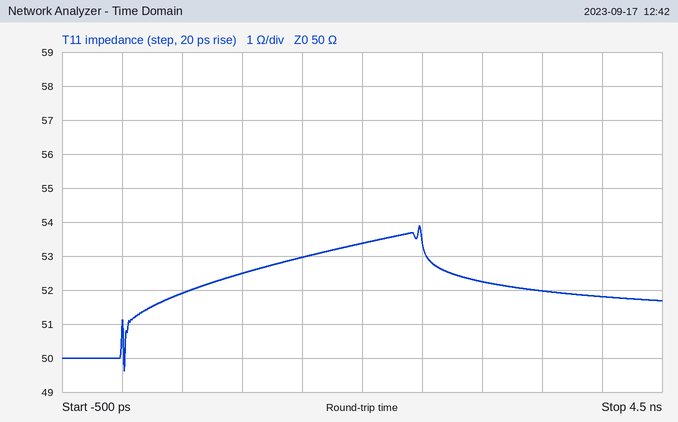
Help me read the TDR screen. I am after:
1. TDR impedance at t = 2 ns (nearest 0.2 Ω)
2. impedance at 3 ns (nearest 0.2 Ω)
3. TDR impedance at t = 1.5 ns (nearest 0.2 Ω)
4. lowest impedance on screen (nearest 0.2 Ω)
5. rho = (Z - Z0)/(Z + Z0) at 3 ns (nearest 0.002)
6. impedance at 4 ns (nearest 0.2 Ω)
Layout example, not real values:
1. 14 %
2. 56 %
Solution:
1. 53.4 Ω
2. 52.2 Ω
3. 53.0 Ω
4. 49.6 Ω
5. +0.022
6. 51.8 Ω
